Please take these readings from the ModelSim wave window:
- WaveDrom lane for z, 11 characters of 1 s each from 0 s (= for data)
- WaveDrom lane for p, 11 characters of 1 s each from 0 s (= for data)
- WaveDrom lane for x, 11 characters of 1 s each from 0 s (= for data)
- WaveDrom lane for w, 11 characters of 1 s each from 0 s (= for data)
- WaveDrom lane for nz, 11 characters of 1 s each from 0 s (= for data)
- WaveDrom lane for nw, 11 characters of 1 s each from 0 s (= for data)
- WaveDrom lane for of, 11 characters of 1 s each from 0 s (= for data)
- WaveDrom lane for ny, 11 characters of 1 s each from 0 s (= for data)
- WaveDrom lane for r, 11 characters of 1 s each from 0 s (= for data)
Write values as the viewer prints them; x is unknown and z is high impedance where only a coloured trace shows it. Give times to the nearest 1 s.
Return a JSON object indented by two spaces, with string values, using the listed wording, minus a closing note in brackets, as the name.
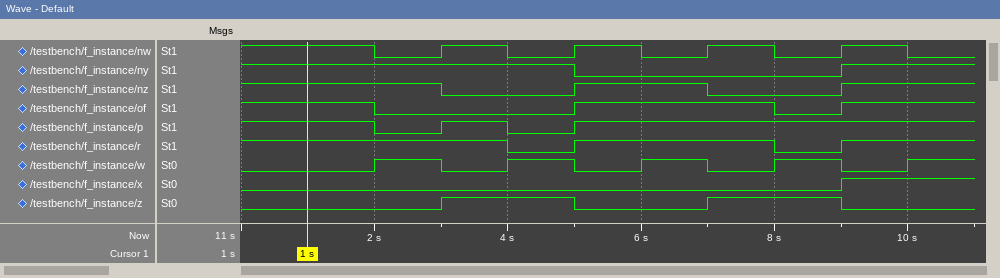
{
  "WaveDrom lane for z, 11 characters of 1 s each from 0 s": "{name: 'z', wave: '0..1.0.1.0.'}",
  "WaveDrom lane for p, 11 characters of 1 s each from 0 s": "{name: 'p', wave: '1.0101.....'}",
  "WaveDrom lane for x, 11 characters of 1 s each from 0 s": "{name: 'x', wave: '0........1.'}",
  "WaveDrom lane for w, 11 characters of 1 s each from 0 s": "{name: 'w', wave: '0.101010101'}",
  "WaveDrom lane for nz, 11 characters of 1 s each from 0 s": "{name: 'nz', wave: '1..0.1.0.1.'}",
  "WaveDrom lane for nw, 11 characters of 1 s each from 0 s": "{name: 'nw', wave: '1.010101010'}",
  "WaveDrom lane for of, 11 characters of 1 s each from 0 s": "{name: 'of', wave: '1.0..1..01.'}",
  "WaveDrom lane for ny, 11 characters of 1 s each from 0 s": "{name: 'ny', wave: '1....0...1.'}",
  "WaveDrom lane for r, 11 characters of 1 s each from 0 s": "{name: 'r', wave: '1...01..01.'}"
}
